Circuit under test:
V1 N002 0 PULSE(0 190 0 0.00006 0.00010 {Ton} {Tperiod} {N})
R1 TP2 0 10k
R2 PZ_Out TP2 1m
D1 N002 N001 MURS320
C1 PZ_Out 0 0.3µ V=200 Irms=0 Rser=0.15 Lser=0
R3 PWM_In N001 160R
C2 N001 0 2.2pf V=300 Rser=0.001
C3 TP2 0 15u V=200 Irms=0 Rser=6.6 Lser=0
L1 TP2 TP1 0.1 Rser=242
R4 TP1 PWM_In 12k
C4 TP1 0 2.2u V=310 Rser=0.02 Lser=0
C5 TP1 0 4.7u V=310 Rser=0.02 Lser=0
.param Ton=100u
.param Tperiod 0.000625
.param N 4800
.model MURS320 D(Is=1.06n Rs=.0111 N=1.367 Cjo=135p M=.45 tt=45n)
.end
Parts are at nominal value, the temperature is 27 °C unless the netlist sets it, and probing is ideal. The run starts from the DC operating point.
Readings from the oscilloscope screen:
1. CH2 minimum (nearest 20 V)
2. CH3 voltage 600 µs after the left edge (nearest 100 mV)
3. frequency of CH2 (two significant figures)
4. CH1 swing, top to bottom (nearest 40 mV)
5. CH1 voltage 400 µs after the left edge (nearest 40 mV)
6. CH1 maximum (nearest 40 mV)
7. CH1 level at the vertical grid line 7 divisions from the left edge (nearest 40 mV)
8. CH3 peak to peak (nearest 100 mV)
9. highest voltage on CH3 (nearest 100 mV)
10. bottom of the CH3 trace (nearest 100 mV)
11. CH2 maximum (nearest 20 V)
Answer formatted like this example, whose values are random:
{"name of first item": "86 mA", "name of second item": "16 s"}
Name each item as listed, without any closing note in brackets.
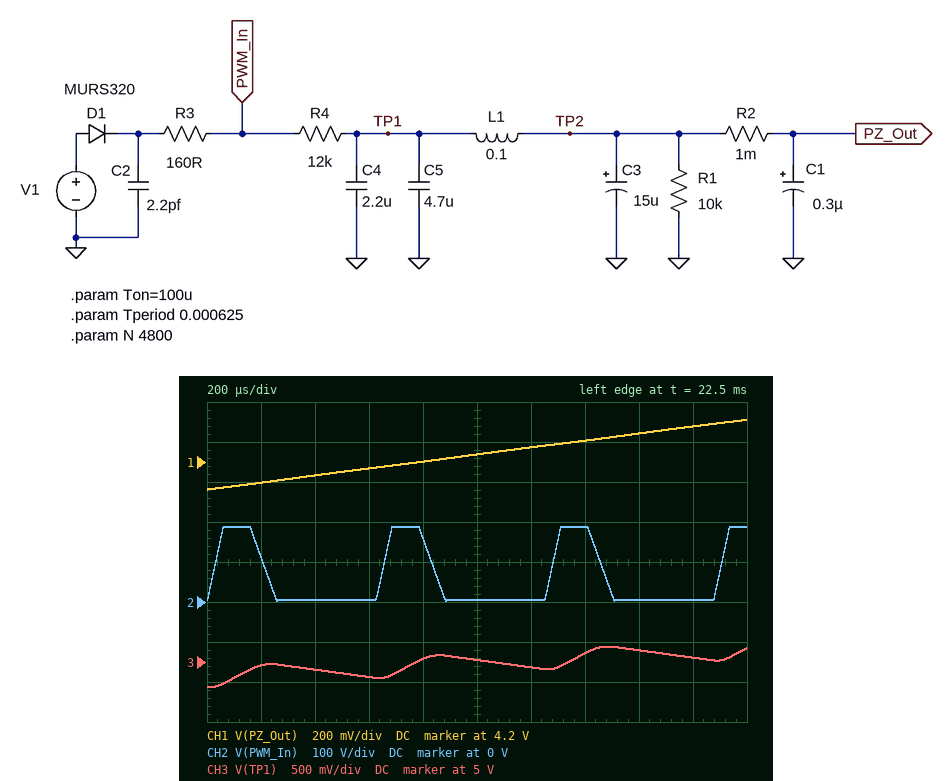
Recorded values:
{"CH2 minimum": "0 V", "CH3 voltage 600 µs after the left edge": "4.8 V", "frequency of CH2": "1.6 kHz", "CH1 swing, top to bottom": "360 mV", "CH1 voltage 400 µs after the left edge": "4.12 V", "CH1 maximum": "4.40 V", "CH1 level at the vertical grid line 7 divisions from the left edge": "4.32 V", "CH3 peak to peak": "500 mV", "highest voltage on CH3": "5.2 V", "bottom of the CH3 trace": "4.7 V", "CH2 maximum": "180 V"}
